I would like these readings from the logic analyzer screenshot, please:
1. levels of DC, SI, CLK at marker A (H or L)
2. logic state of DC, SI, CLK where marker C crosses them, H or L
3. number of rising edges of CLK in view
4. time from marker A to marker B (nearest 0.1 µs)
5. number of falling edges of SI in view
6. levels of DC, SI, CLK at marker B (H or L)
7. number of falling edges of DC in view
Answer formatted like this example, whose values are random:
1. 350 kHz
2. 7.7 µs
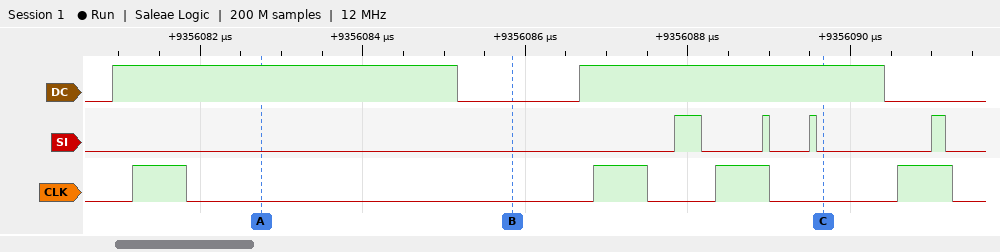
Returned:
1. DC=H, SI=L, CLK=L
2. DC=H, SI=L, CLK=L
3. 4
4. 3.1 µs
5. 4
6. DC=L, SI=L, CLK=L
7. 2
